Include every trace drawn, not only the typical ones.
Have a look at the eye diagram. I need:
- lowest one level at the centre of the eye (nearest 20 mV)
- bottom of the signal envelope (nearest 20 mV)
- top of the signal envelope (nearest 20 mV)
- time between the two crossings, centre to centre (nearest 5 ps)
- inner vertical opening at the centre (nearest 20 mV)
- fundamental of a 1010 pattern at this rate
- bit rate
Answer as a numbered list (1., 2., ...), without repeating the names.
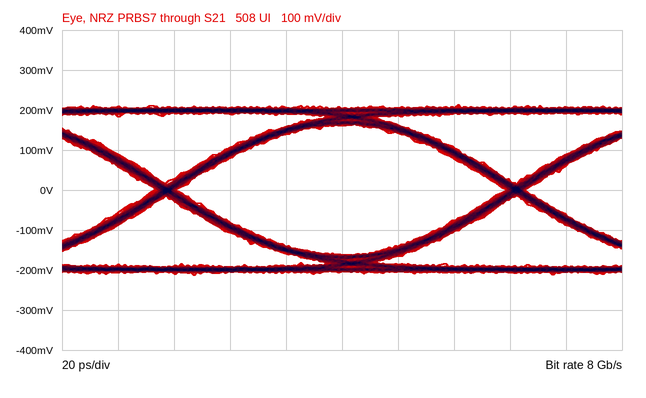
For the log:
1. 160 mV
2. -220 mV
3. 220 mV
4. 125 ps
5. 320 mV
6. 4 GHz
7. 8 Gb/s
